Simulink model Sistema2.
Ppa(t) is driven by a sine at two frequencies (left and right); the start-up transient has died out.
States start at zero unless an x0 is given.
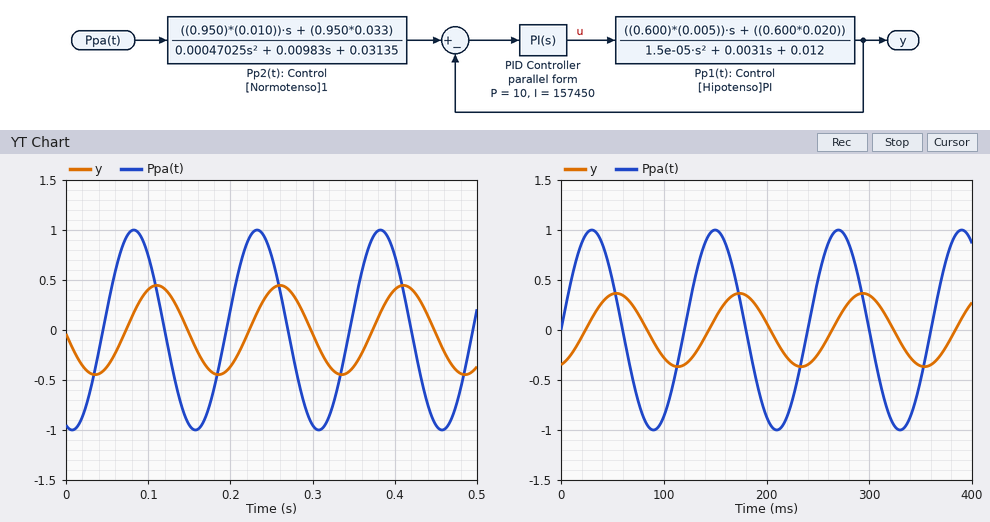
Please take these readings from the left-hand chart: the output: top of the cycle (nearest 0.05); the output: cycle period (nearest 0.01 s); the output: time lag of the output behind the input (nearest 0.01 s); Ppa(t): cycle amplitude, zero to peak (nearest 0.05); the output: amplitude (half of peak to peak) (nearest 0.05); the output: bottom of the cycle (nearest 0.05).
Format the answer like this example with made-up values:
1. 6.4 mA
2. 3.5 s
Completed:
1. 0.45
2. 0.15 s
3. 0.03 s
4. 1.00
5. 0.45
6. -0.45
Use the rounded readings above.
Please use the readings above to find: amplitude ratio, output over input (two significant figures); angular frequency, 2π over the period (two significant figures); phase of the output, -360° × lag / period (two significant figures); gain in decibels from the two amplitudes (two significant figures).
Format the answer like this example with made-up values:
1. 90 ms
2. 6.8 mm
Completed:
1. 0.45
2. 42 rad/s
3. -72°
4. -6.9 dB
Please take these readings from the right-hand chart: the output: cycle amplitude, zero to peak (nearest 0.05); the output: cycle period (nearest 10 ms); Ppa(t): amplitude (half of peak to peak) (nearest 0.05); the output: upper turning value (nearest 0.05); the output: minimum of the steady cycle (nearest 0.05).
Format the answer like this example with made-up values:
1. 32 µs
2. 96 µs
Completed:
1. 0.35
2. 120 ms
3. 1.00
4. 0.35
5. -0.35
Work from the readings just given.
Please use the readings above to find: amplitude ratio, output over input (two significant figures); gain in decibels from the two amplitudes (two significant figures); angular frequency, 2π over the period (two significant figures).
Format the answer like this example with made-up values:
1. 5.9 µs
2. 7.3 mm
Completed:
1. 0.35
2. -9.1 dB
3. 0.052 rad/ms
